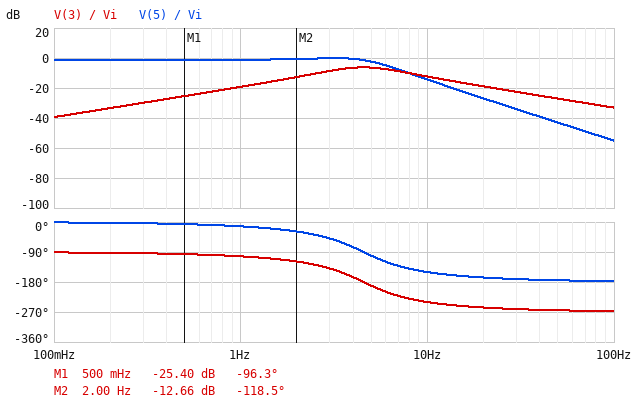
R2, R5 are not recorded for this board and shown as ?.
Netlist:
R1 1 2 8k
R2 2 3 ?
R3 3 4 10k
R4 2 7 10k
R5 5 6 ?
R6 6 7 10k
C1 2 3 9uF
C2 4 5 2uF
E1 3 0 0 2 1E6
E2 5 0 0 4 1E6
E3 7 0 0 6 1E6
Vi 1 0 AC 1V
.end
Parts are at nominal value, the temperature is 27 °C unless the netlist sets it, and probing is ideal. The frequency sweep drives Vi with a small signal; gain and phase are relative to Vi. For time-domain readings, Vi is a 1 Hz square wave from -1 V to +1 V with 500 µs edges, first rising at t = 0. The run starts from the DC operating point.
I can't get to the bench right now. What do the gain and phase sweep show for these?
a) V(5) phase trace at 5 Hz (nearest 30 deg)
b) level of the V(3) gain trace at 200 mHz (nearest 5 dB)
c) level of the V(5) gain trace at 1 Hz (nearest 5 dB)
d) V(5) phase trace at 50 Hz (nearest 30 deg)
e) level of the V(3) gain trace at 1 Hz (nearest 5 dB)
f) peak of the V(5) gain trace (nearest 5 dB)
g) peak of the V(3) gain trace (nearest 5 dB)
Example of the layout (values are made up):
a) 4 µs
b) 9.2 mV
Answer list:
a) -90 deg
b) -35 dB
c) 0 dB
d) -180 deg
e) -20 dB
f) 0 dB
g) -5 dB
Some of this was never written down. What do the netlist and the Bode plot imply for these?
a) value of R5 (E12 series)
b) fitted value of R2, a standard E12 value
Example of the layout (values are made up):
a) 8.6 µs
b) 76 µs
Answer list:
a) 6.8 kΩ
b) 3.9 kΩ
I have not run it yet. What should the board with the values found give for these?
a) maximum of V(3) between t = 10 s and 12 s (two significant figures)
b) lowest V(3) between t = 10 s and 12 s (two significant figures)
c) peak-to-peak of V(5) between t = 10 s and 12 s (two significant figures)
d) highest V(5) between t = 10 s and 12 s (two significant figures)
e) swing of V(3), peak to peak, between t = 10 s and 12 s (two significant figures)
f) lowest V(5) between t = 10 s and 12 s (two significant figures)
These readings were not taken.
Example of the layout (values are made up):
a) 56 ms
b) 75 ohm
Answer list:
a) 530 mV
b) -530 mV
c) 2.3 V
d) 1.1 V
e) 1.1 V
f) -1.1 V
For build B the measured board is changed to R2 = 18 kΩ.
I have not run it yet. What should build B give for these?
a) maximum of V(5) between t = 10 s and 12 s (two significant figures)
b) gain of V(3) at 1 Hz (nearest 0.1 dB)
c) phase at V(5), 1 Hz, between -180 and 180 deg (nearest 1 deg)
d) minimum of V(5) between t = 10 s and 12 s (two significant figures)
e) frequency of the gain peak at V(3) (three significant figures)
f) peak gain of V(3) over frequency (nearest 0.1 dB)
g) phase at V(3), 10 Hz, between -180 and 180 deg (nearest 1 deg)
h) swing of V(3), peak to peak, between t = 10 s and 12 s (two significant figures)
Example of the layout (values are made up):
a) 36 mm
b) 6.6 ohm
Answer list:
a) 2.0 V
b) -19.0 dB
c) -3 deg
d) -2.0 V
e) 4.55 Hz
f) 7.0 dB
g) 97 deg
h) 1.6 V
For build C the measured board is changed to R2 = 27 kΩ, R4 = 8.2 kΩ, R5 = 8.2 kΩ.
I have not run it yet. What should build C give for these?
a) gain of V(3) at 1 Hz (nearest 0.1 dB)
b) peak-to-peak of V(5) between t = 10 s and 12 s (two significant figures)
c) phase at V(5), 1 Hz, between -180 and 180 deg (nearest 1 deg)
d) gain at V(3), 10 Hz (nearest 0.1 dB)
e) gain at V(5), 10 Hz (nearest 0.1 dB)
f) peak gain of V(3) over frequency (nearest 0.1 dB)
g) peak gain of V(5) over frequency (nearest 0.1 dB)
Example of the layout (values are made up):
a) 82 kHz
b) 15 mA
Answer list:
a) -19.1 dB
b) 4.3 V
c) -2 deg
d) -11.1 dB
e) -13.1 dB
f) 10.6 dB
g) 15.4 dB
